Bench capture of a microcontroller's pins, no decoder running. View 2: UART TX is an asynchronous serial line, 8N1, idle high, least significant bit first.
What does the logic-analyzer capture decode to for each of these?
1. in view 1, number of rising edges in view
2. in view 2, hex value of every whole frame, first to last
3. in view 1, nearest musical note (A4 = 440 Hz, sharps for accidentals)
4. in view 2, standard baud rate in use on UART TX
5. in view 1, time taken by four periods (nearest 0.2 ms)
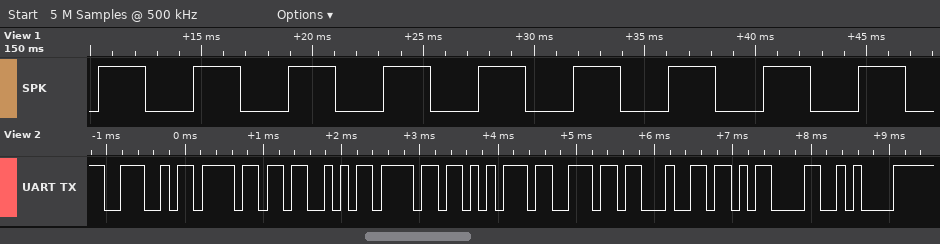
9
4E 6F 53 6F 75 6E 64 0D 0A
A#3
9600 baud
17.2 ms
